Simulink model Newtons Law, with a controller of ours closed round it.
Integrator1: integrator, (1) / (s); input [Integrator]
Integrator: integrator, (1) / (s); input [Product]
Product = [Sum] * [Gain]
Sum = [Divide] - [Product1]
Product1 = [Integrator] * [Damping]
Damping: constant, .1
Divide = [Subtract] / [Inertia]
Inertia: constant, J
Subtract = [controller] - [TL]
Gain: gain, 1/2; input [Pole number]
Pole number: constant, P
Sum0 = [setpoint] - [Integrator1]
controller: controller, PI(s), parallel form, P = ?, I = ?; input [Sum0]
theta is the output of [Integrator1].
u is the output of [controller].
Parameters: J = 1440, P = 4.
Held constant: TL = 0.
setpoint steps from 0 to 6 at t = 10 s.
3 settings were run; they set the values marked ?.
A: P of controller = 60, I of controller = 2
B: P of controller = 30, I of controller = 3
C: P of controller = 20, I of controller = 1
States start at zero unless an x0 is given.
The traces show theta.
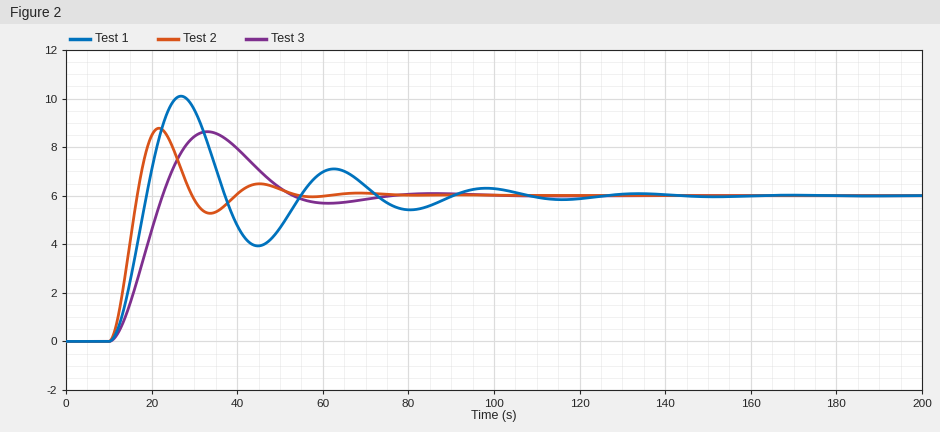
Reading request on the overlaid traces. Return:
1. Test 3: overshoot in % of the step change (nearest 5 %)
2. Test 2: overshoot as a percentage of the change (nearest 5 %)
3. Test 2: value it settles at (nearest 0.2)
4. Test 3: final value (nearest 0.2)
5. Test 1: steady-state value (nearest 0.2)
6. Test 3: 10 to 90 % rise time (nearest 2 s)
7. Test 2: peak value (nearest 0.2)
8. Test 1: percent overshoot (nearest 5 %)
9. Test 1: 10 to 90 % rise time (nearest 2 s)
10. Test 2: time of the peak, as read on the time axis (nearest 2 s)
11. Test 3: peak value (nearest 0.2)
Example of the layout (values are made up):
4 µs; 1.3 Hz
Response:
45 %; 45 %; 6.0; 6.0; 6.0; 8 s; 8.8; 70 %; 6 s; 22 s; 8.6
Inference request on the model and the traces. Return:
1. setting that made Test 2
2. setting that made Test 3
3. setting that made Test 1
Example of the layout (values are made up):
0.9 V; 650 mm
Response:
A; C; B
